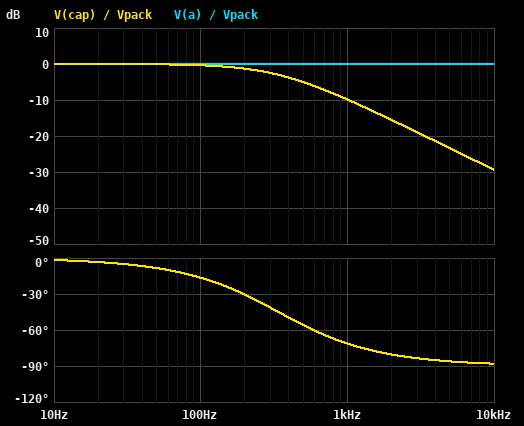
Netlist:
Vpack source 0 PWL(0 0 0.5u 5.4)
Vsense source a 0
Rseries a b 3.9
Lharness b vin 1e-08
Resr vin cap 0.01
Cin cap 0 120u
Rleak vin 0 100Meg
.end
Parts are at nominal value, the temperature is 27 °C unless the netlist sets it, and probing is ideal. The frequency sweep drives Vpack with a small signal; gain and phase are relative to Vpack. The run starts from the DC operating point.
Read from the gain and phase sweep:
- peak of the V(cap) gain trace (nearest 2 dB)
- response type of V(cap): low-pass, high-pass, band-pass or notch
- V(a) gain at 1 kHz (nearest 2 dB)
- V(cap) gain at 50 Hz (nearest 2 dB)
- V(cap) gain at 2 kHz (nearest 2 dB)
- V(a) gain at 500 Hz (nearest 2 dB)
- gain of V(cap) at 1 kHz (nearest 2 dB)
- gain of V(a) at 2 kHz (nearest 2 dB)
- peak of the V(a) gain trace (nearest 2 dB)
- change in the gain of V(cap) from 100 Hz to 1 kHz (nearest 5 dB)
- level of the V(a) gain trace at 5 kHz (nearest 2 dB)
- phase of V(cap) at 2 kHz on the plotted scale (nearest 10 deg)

0 dB
low-pass
0 dB
0 dB
-16 dB
0 dB
-10 dB
0 dB
0 dB
-10 dB
0 dB
-80 deg
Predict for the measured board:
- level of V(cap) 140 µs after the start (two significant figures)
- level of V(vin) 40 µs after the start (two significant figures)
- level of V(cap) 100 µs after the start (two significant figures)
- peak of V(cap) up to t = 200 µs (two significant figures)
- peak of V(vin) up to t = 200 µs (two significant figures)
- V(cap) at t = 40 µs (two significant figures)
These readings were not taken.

1.4 V
450 mV
1.0 V
1.9 V
1.9 V
440 mV
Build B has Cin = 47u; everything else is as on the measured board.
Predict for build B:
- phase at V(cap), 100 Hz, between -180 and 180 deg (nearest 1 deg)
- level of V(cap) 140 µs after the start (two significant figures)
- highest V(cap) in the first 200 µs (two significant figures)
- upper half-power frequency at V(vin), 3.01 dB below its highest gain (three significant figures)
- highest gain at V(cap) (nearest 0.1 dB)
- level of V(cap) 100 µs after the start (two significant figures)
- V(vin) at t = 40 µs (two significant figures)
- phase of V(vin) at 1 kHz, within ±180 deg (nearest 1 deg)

-7 deg
2.9 V
3.6 V
866 Hz
0 dB
2.3 V
1.1 V
-49 deg
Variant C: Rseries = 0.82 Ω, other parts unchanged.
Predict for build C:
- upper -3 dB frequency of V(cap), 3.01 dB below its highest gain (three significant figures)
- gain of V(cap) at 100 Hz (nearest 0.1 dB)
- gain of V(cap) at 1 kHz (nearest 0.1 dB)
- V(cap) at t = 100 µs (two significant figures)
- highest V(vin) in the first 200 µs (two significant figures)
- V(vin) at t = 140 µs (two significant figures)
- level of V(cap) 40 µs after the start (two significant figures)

1.60 kHz
0 dB
-1.4 dB
3.4 V
4.7 V
4.1 V
1.8 V
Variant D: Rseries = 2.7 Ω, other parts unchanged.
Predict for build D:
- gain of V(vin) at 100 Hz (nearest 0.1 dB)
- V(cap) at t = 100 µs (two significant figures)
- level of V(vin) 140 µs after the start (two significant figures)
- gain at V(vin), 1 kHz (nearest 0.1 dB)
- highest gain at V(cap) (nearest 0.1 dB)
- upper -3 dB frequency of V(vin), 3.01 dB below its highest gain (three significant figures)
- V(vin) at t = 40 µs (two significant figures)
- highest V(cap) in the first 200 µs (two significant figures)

-0.2 dB
1.4 V
1.9 V
-7.1 dB
0 dB
489 Hz
640 mV
2.5 V
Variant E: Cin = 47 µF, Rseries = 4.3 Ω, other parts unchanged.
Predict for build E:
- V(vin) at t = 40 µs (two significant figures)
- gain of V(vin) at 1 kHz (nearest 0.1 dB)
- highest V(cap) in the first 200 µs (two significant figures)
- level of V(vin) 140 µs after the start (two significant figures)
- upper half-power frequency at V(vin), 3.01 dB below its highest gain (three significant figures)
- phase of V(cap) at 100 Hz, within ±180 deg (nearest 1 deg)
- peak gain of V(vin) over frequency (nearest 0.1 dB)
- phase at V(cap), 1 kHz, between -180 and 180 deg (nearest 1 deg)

970 mV
-4.2 dB
3.4 V
2.7 V
786 Hz
-7 deg
0 dB
-52 deg
